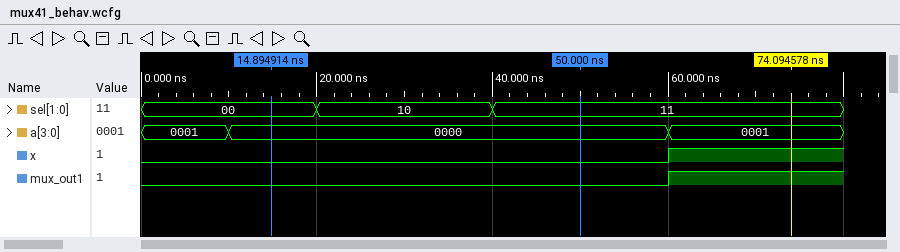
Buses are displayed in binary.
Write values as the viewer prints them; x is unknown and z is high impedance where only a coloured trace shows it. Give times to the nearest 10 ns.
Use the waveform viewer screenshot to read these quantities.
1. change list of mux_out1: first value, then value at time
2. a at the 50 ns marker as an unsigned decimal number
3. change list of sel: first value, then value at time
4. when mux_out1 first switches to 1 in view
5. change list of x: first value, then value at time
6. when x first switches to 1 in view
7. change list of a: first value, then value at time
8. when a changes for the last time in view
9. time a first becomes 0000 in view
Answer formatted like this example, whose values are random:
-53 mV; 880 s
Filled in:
0, 1 at 60 ns; 0; 00, 10 at 20 ns, 11 at 40 ns; 60 ns; 0, 1 at 60 ns; 60 ns; 0001, 0000 at 10 ns, 0001 at 60 ns; 60 ns; 10 ns
